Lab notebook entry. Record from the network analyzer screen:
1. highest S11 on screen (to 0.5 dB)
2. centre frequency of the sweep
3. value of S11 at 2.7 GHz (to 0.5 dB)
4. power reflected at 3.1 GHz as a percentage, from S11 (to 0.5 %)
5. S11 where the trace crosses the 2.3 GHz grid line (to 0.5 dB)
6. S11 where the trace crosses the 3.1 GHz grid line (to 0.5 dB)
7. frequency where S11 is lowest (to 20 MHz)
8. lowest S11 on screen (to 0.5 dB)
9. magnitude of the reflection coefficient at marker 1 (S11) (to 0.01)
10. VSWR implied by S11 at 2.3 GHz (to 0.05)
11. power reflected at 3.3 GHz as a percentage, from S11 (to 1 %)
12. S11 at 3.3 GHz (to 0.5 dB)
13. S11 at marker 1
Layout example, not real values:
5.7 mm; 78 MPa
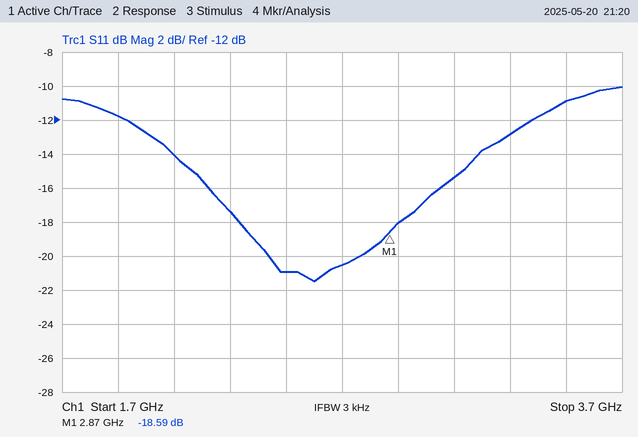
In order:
-10.0 dB; 2.7 GHz; -20.5 dB; 3.0 %; -17.5 dB; -15.5 dB; 2.60 GHz; -21.5 dB; 0.12; 1.30; 5 %; -13.0 dB; -18.59 dB
